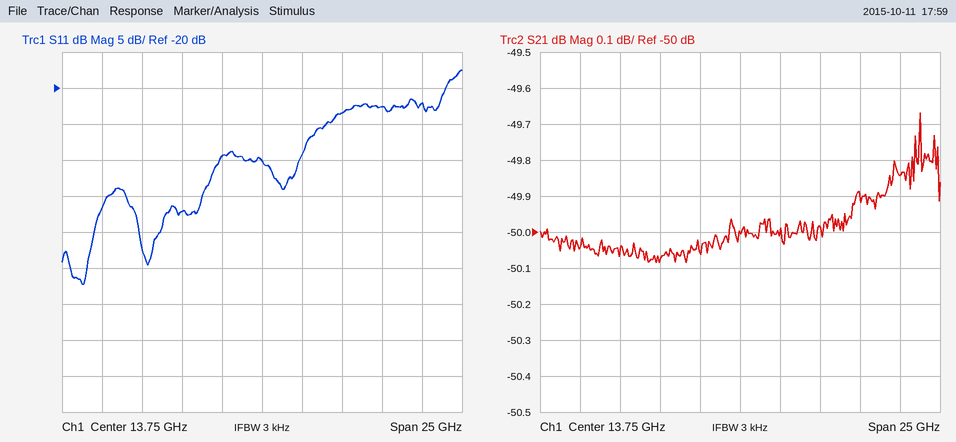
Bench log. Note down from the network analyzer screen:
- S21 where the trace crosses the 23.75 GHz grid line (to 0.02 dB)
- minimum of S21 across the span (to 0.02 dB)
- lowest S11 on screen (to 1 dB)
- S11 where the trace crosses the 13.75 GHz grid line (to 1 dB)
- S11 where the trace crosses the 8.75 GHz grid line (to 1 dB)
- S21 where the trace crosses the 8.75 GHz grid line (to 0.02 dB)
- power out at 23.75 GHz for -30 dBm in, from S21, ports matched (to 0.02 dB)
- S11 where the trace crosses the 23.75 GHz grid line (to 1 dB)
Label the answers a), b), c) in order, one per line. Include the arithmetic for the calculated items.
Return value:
a) -49.84 dB
b) -50.08 dB
c) -47 dB
d) -30 dB
e) -37 dB
f) -50.08 dB
g) -30 dBm + (-49.84 dB) = -79.84 dBm
h) -22 dB
